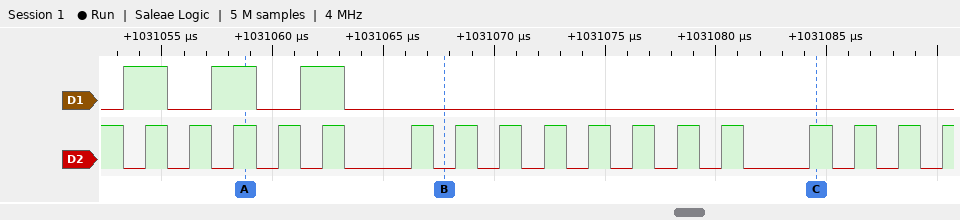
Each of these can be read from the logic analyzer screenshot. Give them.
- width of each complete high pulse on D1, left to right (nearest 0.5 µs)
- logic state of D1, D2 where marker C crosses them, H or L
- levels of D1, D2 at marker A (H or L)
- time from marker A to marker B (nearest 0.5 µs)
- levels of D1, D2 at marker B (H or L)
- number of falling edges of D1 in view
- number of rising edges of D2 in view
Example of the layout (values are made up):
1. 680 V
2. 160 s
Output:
1. 2 µs, 2 µs, 2 µs
2. D1=L, D2=H
3. D1=H, D2=H
4. 9 µs
5. D1=L, D2=L
6. 3
7. 17
